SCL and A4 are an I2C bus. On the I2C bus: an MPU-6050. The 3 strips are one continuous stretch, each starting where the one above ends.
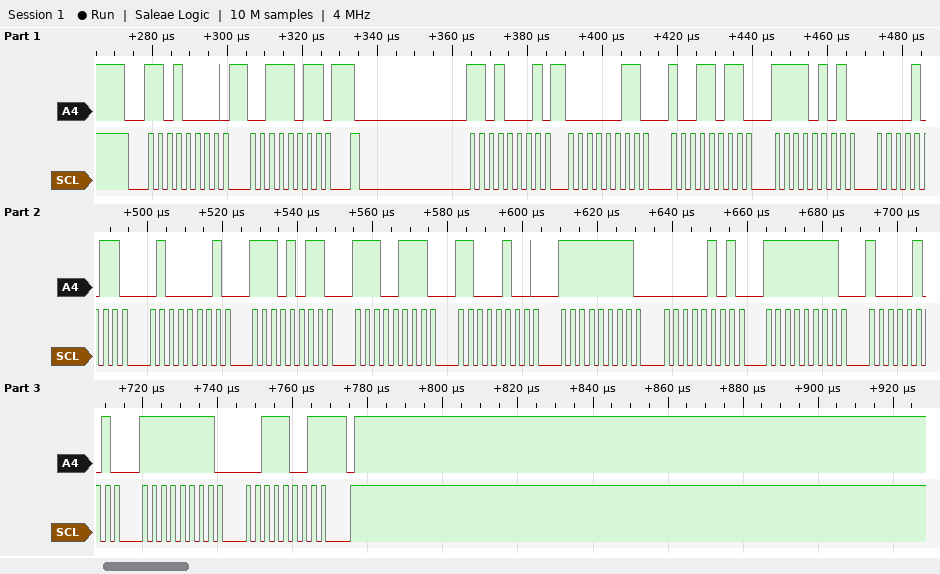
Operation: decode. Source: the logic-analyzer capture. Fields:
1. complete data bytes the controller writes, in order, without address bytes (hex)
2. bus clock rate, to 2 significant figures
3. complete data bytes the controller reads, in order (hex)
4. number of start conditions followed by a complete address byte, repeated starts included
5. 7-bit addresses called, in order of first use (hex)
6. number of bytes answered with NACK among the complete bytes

3B
400 kHz
03 9B F5 0B 41 EB E7 C4 FF 05 FF 85 FF 39
2
0x68
1
